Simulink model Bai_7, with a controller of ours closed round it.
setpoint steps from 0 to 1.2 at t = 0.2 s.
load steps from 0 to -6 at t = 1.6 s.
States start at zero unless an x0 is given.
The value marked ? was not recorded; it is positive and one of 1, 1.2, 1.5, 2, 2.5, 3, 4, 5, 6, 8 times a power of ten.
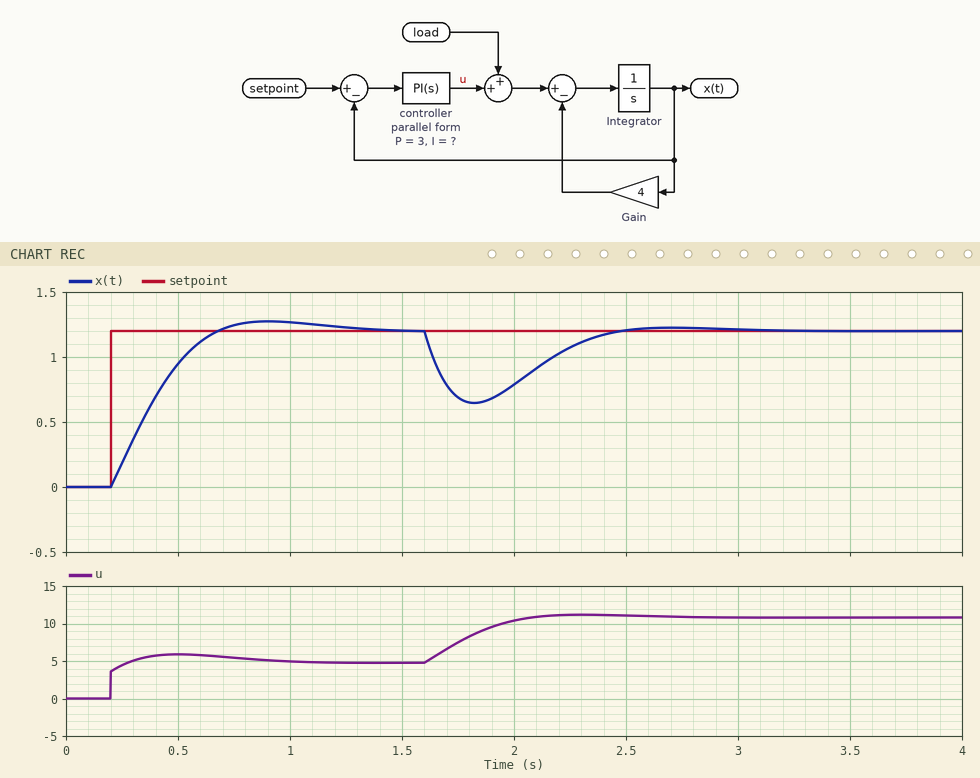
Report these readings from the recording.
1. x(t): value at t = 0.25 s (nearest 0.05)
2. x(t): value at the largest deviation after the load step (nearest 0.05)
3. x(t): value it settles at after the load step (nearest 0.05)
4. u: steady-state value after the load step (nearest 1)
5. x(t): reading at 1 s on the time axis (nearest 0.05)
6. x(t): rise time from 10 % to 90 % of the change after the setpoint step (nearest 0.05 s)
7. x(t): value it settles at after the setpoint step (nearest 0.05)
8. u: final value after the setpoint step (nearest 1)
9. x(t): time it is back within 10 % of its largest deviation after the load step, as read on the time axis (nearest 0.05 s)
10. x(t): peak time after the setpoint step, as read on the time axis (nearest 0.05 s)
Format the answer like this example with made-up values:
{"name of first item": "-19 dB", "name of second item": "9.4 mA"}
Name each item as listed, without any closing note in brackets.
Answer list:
{"x(t): value at t = 0.25 s": "0.20", "x(t): value at the largest deviation after the load step": "0.65", "x(t): value it settles at after the load step": "1.20", "u: steady-state value after the load step": "11", "x(t): reading at 1 s on the time axis": "1.25", "x(t): rise time from 10 % to 90 % of the change after the setpoint step": "0.35 s", "x(t): value it settles at after the setpoint step": "1.20", "u: final value after the setpoint step": "5", "x(t): time it is back within 10 % of its largest deviation after the load step, as read on the time axis": "2.35 s", "x(t): peak time after the setpoint step, as read on the time axis": "0.90 s"}
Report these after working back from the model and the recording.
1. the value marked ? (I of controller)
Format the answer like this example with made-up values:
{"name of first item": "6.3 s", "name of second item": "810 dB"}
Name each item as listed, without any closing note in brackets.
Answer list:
{"the value marked ?": "25"}
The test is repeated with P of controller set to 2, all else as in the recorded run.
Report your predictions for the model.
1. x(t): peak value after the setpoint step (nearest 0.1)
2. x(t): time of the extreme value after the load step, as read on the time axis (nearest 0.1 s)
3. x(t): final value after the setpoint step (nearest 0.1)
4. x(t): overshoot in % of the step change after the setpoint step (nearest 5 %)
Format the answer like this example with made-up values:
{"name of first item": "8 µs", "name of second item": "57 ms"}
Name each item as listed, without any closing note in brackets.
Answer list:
{"x(t): peak value after the setpoint step": "1.3", "x(t): time of the extreme value after the load step, as read on the time axis": "1.8 s", "x(t): final value after the setpoint step": "1.2", "x(t): overshoot in % of the step change after the setpoint step": "10 %"}
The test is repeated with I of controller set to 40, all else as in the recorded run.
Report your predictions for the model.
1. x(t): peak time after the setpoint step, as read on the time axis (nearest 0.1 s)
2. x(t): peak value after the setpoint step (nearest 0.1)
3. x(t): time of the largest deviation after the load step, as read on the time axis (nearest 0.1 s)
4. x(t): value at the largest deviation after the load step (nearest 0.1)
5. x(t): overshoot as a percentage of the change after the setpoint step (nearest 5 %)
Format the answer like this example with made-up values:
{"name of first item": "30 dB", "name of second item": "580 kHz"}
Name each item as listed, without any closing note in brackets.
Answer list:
{"x(t): peak time after the setpoint step, as read on the time axis": "0.7 s", "x(t): peak value after the setpoint step": "1.4", "x(t): time of the largest deviation after the load step, as read on the time axis": "1.8 s", "x(t): value at the largest deviation after the load step": "0.7", "x(t): overshoot as a percentage of the change after the setpoint step": "15 %"}
